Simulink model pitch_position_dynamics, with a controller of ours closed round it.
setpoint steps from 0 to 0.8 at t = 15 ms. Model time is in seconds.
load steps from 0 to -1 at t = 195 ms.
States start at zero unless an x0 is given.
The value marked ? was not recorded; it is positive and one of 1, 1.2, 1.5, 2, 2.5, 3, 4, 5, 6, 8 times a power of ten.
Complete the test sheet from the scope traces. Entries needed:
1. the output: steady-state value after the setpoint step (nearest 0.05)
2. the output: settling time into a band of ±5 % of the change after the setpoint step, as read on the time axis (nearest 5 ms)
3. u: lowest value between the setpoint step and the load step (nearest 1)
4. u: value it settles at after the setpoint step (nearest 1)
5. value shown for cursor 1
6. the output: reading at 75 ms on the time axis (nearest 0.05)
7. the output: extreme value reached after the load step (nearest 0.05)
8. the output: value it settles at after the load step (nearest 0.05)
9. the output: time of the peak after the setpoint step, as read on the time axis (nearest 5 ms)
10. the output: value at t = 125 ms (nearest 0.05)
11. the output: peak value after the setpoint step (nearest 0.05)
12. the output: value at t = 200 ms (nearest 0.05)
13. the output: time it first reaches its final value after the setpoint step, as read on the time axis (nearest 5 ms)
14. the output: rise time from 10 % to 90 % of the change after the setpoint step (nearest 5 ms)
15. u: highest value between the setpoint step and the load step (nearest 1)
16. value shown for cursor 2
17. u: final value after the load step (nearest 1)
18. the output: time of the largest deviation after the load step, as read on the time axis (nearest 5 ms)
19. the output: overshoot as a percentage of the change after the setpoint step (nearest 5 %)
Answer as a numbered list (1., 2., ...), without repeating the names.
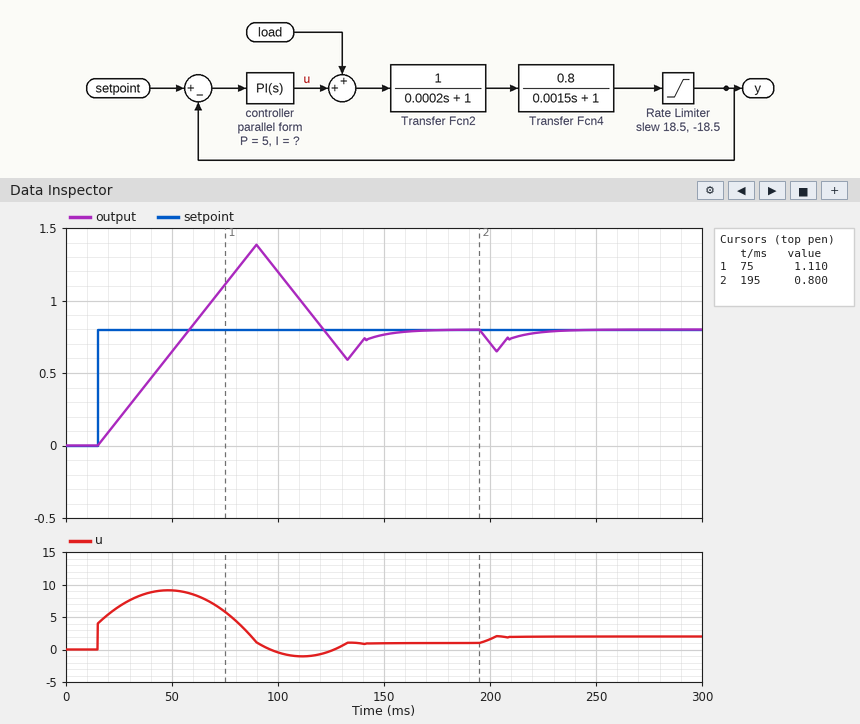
1. 0.80
2. 150 ms
3. -1
4. 1
5. 1.110
6. 1.10
7. 0.65
8. 0.80
9. 90 ms
10. 0.75
11. 1.40
12. 0.70
13. 60 ms
14. 35 ms
15. 9
16. 0.800
17. 2
18. 205 ms
19. 75 %
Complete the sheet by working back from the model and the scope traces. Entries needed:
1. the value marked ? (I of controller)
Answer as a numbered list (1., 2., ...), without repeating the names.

1. 500
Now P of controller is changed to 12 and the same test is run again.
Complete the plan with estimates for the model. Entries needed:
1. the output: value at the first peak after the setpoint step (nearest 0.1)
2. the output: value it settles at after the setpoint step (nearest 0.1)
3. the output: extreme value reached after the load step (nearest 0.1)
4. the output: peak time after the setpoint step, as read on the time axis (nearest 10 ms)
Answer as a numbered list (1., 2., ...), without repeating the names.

1. 1.2
2. 0.8
3. 0.7
4. 80 ms
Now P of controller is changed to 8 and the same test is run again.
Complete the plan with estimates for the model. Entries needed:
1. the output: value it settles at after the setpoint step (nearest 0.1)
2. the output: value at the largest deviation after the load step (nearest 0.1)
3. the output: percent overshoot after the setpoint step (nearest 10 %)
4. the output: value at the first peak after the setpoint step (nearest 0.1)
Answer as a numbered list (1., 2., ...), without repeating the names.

1. 0.8
2. 0.7
3. 60 %
4. 1.3
